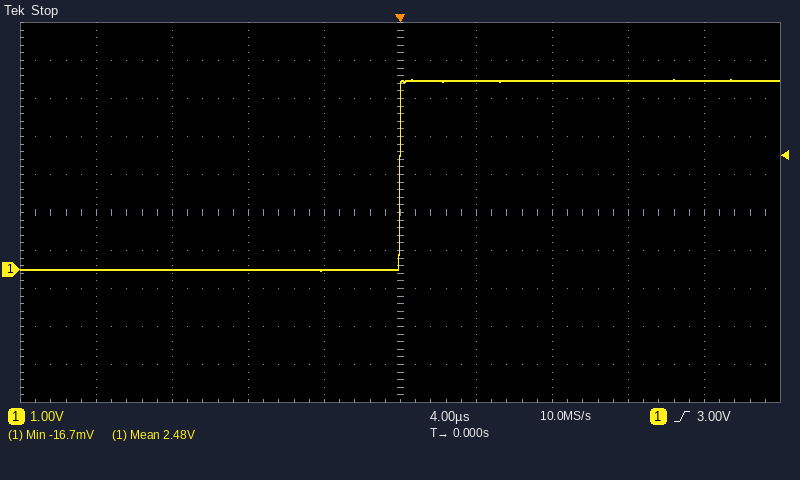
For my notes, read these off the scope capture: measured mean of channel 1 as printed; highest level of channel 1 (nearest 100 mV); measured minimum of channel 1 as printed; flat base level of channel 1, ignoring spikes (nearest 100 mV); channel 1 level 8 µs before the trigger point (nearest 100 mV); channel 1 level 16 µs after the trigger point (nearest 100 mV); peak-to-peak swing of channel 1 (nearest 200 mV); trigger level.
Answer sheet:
2.48 V
5.0 V
-16.7 mV
0.0 V
0.0 V
5.0 V
5.0 V
3.00 V
